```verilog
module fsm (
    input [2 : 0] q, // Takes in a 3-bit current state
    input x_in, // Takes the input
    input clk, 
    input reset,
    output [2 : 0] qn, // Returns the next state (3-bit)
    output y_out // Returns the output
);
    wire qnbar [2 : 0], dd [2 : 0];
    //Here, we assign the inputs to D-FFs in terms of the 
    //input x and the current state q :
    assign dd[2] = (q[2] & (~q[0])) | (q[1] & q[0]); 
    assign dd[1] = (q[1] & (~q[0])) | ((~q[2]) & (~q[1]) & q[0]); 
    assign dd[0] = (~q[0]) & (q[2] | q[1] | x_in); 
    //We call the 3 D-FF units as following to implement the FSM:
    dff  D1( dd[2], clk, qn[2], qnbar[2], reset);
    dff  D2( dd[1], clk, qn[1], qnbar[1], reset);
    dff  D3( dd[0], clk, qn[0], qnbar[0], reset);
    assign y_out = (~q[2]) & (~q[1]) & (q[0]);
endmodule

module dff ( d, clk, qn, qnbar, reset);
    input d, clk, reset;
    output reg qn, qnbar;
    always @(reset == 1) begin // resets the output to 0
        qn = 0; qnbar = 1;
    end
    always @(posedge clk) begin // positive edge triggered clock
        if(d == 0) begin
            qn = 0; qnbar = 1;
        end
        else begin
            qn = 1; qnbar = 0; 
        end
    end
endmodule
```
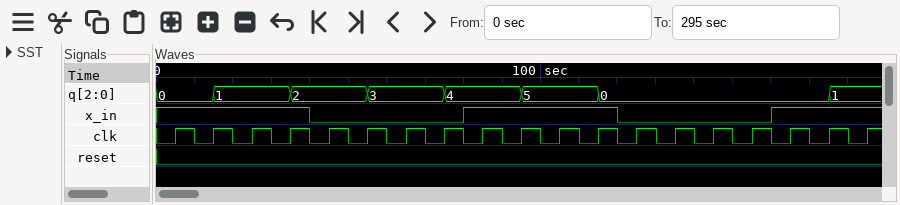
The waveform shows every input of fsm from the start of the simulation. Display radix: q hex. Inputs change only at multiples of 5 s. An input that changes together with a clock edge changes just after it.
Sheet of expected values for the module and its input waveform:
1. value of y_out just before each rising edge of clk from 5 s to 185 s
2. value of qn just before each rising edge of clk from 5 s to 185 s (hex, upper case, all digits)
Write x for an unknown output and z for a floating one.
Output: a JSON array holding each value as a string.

["0 0 1 1 0 0 0 0 0 0 0 0 0 0 0 0 0 0 1", "0, 1, 1, 2, 2, 3, 3, 4, 4, 5, 5, 0, 0, 0, 0, 0, 0, 1, 1"]
